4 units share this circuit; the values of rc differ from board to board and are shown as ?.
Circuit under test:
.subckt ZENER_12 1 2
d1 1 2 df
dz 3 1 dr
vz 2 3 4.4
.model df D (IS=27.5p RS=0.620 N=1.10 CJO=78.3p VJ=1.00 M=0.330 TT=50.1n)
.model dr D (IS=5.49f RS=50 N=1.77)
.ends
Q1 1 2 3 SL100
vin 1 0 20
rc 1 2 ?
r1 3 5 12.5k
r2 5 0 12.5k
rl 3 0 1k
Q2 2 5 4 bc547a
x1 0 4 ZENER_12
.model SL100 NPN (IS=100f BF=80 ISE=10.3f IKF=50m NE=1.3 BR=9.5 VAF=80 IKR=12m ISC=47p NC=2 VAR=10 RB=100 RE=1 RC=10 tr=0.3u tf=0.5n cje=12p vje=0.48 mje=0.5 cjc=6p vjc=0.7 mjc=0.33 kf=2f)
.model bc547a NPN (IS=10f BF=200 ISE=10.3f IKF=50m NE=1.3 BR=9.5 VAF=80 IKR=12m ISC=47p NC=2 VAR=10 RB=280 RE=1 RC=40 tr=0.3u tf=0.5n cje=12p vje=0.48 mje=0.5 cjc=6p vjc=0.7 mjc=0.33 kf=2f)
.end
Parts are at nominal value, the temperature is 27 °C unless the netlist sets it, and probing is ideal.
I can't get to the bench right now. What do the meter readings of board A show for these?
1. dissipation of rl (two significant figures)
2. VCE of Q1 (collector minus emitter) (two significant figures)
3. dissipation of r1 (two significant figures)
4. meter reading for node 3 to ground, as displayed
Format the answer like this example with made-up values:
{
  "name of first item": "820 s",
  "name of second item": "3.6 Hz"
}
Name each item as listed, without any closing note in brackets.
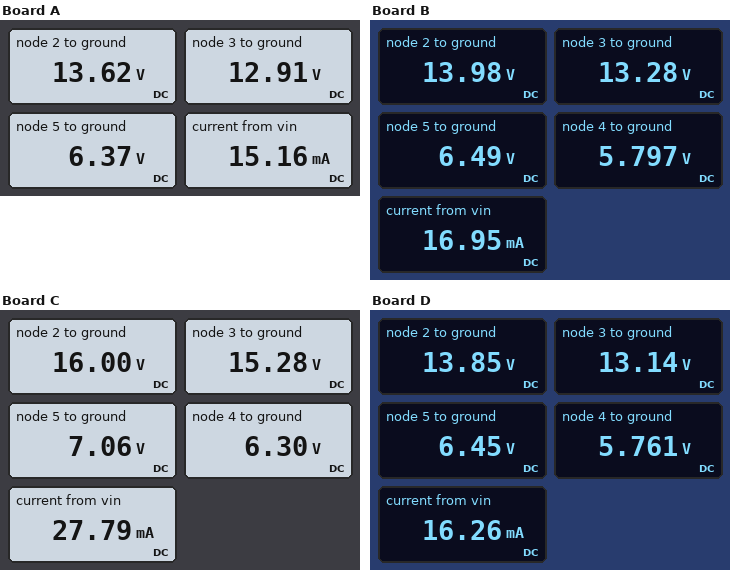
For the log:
{
  "dissipation of rl": "170 mW",
  "VCE of Q1 (collector minus emitter)": "7.1 V",
  "dissipation of r1": "3.4 mW",
  "meter reading for node 3 to ground, as displayed": "12.91 V"
}
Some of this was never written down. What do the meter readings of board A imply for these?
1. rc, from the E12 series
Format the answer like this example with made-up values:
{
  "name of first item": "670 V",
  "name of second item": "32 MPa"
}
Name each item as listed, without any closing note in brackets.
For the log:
{
  "rc, from the E12 series": "3.3 kΩ"
}
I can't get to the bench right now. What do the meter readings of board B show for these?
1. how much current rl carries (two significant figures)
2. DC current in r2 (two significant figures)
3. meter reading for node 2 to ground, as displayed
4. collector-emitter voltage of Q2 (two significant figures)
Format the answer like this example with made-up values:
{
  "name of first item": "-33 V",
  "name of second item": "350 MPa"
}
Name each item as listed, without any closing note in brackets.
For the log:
{
  "how much current rl carries": "13 mA",
  "DC current in r2": "520 µA",
  "meter reading for node 2 to ground, as displayed": "13.98 V",
  "collector-emitter voltage of Q2": "8.2 V"
}
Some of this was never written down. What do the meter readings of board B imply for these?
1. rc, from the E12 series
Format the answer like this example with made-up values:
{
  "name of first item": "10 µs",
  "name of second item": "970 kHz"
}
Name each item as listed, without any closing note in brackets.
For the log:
{
  "rc, from the E12 series": "1.8 kΩ"
}
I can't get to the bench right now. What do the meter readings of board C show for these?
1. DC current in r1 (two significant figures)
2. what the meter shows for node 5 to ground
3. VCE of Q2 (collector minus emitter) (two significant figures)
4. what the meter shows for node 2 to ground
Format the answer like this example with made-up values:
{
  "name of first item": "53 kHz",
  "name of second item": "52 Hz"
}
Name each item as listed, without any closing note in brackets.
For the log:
{
  "DC current in r1": "660 µA",
  "what the meter shows for node 5 to ground": "7.06 V",
  "VCE of Q2 (collector minus emitter)": "9.7 V",
  "what the meter shows for node 2 to ground": "16.00 V"
}
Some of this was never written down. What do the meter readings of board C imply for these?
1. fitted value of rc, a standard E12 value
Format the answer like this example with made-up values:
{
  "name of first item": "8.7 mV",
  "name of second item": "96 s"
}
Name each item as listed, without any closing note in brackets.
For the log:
{
  "fitted value of rc, a standard E12 value": "330 Ω"
}
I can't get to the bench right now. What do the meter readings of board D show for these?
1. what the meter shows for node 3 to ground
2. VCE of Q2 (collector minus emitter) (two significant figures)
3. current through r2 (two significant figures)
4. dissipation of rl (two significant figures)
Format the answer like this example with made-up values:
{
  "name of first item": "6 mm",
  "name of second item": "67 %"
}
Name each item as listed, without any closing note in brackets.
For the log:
{
  "what the meter shows for node 3 to ground": "13.14 V",
  "VCE of Q2 (collector minus emitter)": "8.1 V",
  "current through r2": "520 µA",
  "dissipation of rl": "170 mW"
}
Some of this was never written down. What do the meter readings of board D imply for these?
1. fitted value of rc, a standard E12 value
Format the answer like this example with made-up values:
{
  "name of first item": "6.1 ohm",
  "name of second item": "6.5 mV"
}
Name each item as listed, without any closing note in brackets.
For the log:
{
  "fitted value of rc, a standard E12 value": "2.2 kΩ"
}
